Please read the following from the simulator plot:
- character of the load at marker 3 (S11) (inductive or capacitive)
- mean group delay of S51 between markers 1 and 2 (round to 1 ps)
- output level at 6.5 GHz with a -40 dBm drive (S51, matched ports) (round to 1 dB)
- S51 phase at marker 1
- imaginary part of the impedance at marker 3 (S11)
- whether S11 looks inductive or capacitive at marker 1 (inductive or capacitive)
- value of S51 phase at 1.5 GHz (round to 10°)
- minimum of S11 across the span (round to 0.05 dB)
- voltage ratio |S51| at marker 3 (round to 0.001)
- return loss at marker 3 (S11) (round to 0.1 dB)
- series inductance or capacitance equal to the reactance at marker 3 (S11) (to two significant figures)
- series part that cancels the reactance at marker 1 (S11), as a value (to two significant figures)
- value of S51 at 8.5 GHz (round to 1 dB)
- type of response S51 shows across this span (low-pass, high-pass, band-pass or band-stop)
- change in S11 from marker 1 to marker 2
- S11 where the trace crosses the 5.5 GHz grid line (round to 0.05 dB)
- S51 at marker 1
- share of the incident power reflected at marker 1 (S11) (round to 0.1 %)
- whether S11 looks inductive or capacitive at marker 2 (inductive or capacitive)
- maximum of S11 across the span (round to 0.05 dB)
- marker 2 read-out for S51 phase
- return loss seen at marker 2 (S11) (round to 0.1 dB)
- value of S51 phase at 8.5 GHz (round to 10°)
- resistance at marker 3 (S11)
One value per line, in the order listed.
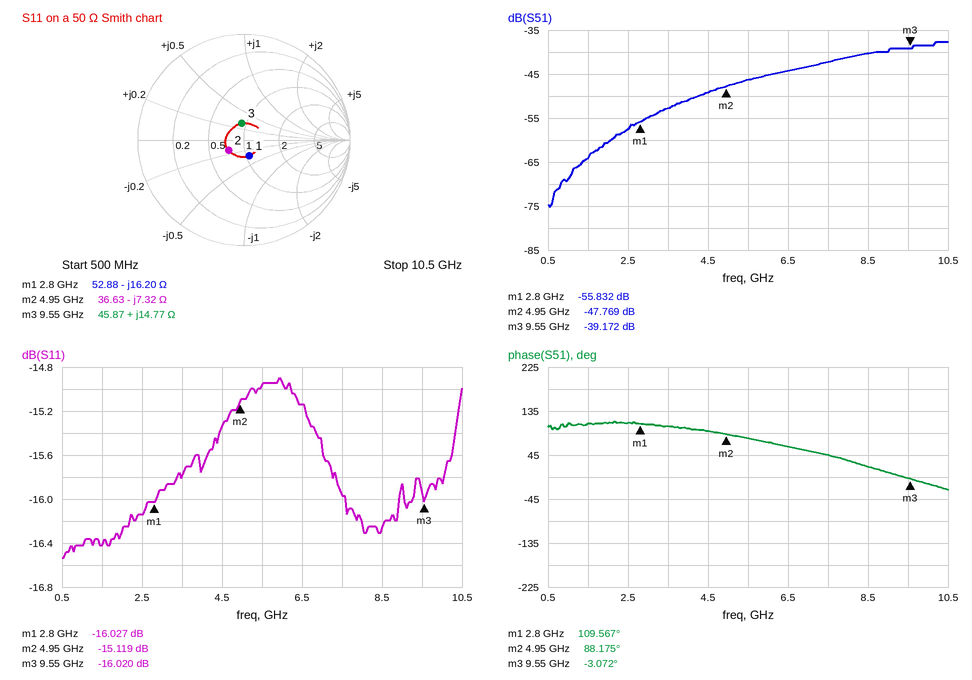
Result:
inductive
28 ps
-84 dBm
109.567°
+14.77 Ω
capacitive
110°
-16.55 dB
0.011
16.0 dB
250 pH
920 pH
-40 dB
high-pass
0.908 dB
-14.95 dB
-55.832 dB
2.5 %
capacitive
-14.90 dB
88.175°
15.1 dB
20°
45.87 Ω
